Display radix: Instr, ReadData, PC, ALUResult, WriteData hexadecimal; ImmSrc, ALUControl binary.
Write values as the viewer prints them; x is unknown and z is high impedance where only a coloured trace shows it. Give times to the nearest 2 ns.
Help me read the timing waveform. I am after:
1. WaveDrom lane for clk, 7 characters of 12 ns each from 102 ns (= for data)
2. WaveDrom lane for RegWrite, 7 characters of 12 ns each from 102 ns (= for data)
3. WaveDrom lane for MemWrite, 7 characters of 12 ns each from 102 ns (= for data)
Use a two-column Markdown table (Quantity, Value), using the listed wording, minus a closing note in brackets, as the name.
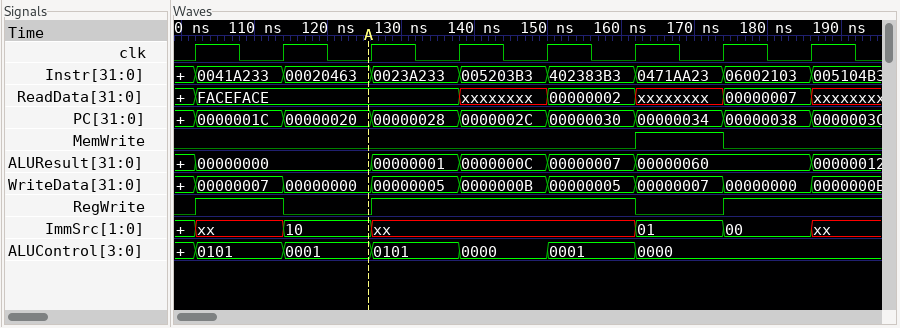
| Quantity | Value |
|---|---|
| WaveDrom lane for clk, 7 characters of 12 ns each from 102 ns | {name: 'clk', wave: 'p......'} |
| WaveDrom lane for RegWrite, 7 characters of 12 ns each from 102 ns | {name: 'RegWrite', wave: '101..01'} |
| WaveDrom lane for MemWrite, 7 characters of 12 ns each from 102 ns | {name: 'MemWrite', wave: '0....10'} |
